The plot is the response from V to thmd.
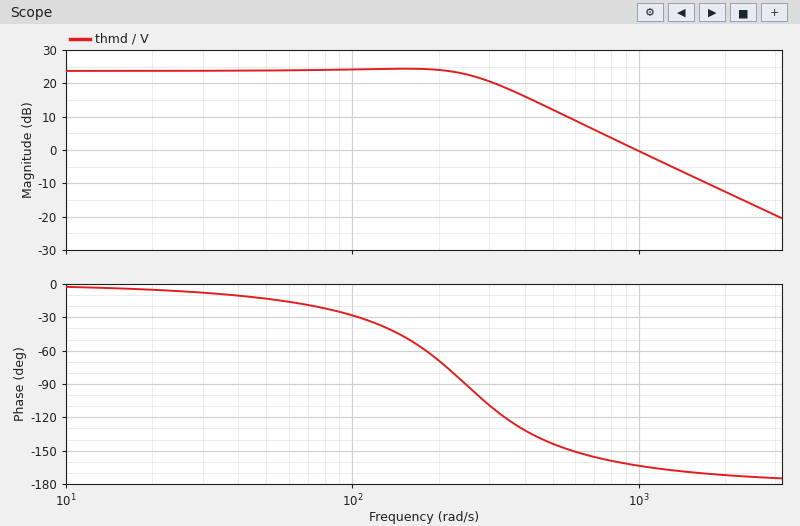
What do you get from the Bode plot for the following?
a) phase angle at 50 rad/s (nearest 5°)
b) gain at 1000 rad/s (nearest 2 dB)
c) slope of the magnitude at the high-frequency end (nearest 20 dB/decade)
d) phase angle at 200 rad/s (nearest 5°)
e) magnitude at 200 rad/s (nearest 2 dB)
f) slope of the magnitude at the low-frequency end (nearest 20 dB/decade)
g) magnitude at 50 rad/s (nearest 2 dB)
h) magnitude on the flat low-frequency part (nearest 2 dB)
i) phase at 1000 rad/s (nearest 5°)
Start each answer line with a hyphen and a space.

- -15°
- 0 dB
- -40 dB/decade
- -70°
- 24 dB
- 0 dB/decade
- 24 dB
- 24 dB
- -165°
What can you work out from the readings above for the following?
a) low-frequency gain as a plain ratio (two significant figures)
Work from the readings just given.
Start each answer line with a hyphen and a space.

- 16
